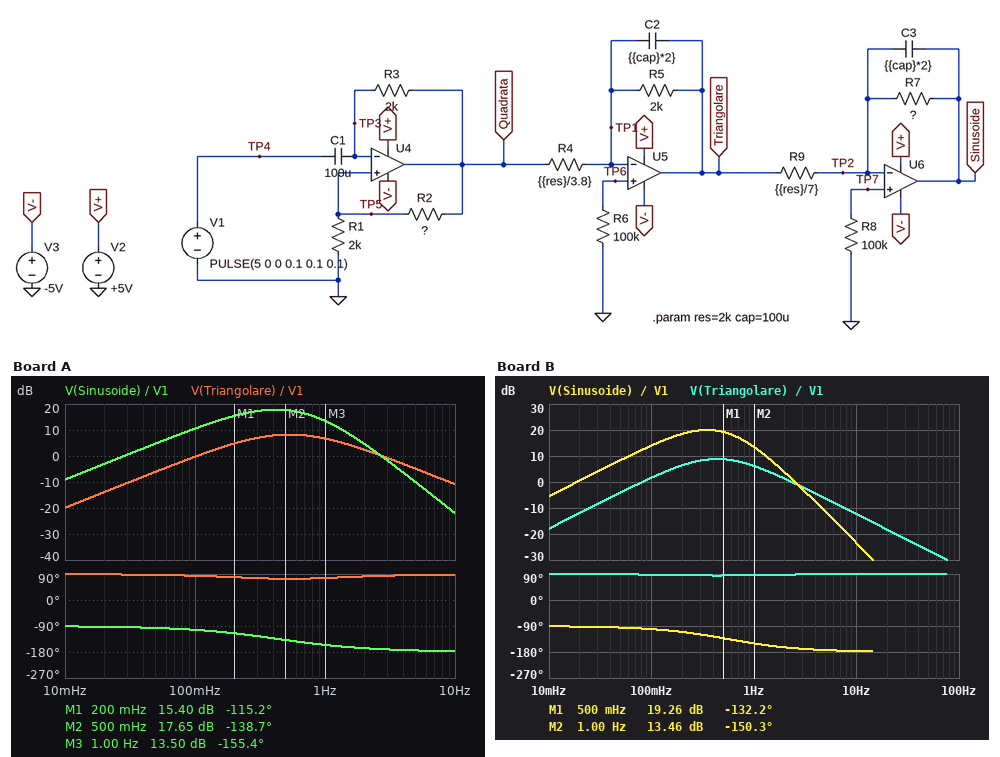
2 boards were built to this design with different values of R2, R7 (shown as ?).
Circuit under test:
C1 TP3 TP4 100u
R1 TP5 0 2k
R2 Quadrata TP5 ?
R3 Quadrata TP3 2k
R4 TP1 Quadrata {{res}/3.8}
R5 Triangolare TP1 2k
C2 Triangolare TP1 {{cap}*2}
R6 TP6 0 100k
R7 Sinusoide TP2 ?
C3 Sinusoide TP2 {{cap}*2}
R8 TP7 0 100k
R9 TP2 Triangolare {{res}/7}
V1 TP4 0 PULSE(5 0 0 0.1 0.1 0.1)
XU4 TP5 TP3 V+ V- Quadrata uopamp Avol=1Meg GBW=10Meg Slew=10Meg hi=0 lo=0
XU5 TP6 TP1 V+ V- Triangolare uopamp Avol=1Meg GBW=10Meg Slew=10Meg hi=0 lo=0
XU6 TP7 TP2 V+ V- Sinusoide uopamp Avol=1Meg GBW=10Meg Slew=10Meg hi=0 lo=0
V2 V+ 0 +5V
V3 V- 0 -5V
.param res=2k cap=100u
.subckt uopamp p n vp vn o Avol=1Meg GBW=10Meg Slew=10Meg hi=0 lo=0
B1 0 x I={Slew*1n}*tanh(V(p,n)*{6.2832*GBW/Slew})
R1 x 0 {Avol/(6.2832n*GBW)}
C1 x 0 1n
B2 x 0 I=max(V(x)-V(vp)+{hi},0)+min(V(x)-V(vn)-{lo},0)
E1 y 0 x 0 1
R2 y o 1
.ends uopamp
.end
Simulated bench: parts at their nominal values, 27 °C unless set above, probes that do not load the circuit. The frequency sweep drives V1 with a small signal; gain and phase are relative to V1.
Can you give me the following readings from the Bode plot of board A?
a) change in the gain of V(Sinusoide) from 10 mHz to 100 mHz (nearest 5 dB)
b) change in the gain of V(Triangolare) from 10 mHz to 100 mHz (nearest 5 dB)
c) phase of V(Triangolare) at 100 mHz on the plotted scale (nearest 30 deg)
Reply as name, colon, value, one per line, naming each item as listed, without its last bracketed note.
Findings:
change in the gain of V(Sinusoide) from 10 mHz to 100 mHz: 20 dB
change in the gain of V(Triangolare) from 10 mHz to 100 mHz: 20 dB
phase of V(Triangolare) at 100 mHz on the plotted scale: 90 deg
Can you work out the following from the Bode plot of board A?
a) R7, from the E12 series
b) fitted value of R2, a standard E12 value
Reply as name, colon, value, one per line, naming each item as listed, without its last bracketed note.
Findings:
R7, from the E12 series: 1 kΩ
fitted value of R2, a standard E12 value: 1.8 kΩ
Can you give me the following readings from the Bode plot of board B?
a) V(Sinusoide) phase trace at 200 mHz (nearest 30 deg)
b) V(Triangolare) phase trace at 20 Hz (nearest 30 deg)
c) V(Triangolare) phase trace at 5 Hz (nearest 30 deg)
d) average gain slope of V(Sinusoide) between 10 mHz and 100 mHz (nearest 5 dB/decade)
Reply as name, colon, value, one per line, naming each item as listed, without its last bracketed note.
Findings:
V(Sinusoide) phase trace at 200 mHz: -120 deg
V(Triangolare) phase trace at 20 Hz: 90 deg
V(Triangolare) phase trace at 5 Hz: 90 deg
average gain slope of V(Sinusoide) between 10 mHz and 100 mHz: 20 dB/decade
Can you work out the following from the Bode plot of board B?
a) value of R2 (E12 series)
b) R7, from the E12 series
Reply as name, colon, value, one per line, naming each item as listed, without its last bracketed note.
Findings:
value of R2: 1.2 kΩ
R7, from the E12 series: 1.2 kΩ
